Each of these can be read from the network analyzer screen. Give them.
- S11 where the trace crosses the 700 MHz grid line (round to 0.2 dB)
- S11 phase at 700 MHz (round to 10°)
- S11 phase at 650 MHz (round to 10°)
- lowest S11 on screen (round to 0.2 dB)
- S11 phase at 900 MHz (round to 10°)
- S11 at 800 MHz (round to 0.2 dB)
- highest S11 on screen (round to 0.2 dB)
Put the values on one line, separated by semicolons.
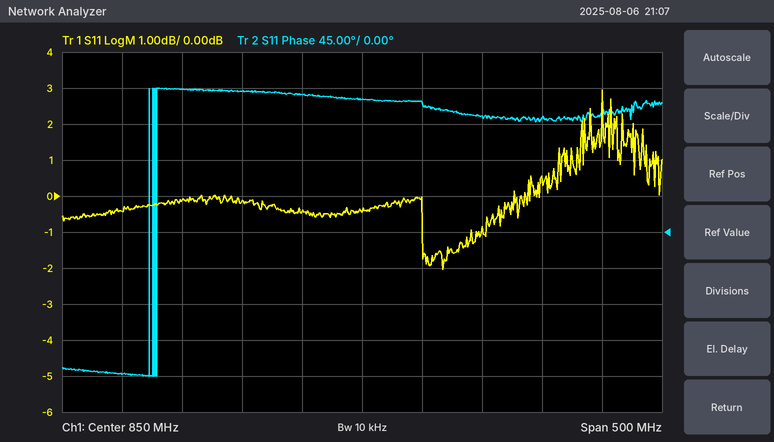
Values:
-0.2 dB; 180°; -180°; -2.0 dB; 160°; -0.4 dB; 3.0 dB
